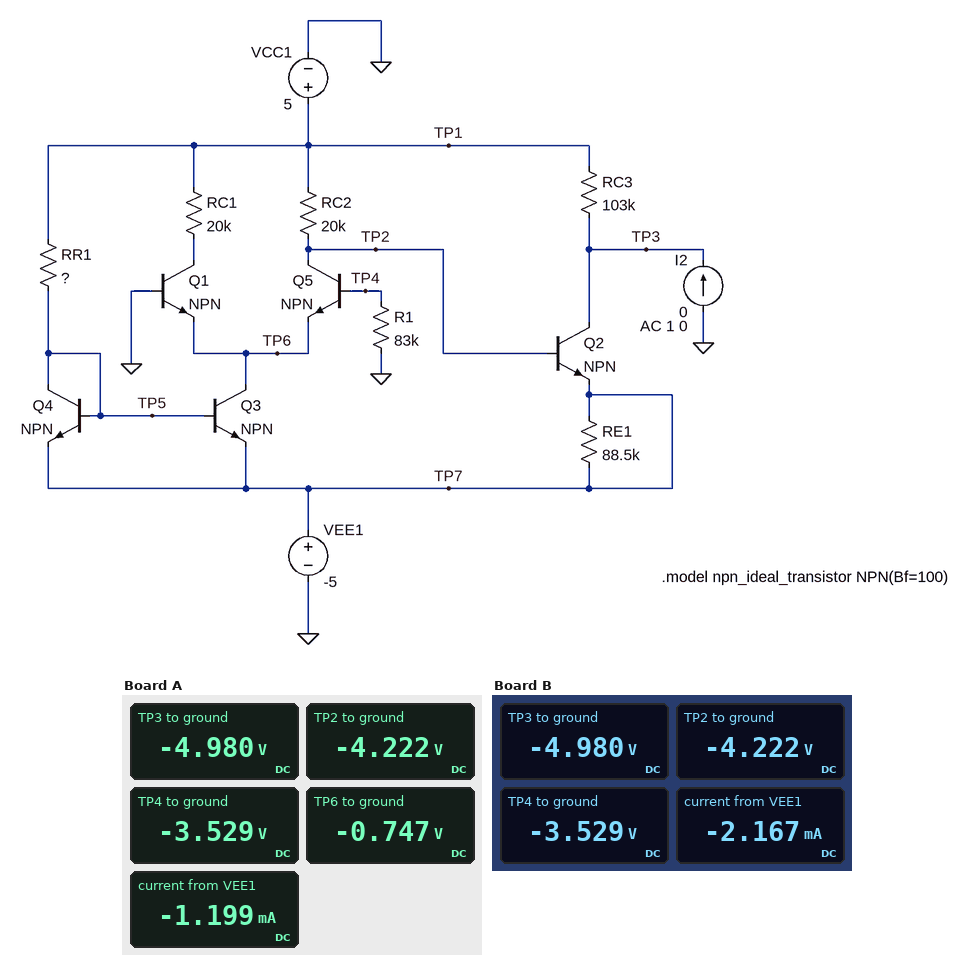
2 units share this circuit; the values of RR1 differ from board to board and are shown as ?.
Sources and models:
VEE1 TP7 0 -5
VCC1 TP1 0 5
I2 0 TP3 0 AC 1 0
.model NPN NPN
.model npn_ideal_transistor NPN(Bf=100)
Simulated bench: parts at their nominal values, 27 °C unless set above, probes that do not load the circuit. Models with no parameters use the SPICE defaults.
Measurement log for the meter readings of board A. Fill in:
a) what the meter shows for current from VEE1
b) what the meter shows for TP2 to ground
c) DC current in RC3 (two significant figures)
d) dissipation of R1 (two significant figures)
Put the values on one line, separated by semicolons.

-1.199 mA; -4.222 V; 97 µA; 150 µW
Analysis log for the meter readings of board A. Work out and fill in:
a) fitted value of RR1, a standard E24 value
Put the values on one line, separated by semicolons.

33 kΩ
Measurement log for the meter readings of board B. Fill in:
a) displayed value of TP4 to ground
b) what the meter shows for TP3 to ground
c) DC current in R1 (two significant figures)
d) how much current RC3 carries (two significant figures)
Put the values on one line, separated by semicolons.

-3.529 V; -4.980 V; 43 µA; 97 µA
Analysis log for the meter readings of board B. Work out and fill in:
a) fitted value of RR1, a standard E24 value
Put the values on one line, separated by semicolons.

12 kΩ
